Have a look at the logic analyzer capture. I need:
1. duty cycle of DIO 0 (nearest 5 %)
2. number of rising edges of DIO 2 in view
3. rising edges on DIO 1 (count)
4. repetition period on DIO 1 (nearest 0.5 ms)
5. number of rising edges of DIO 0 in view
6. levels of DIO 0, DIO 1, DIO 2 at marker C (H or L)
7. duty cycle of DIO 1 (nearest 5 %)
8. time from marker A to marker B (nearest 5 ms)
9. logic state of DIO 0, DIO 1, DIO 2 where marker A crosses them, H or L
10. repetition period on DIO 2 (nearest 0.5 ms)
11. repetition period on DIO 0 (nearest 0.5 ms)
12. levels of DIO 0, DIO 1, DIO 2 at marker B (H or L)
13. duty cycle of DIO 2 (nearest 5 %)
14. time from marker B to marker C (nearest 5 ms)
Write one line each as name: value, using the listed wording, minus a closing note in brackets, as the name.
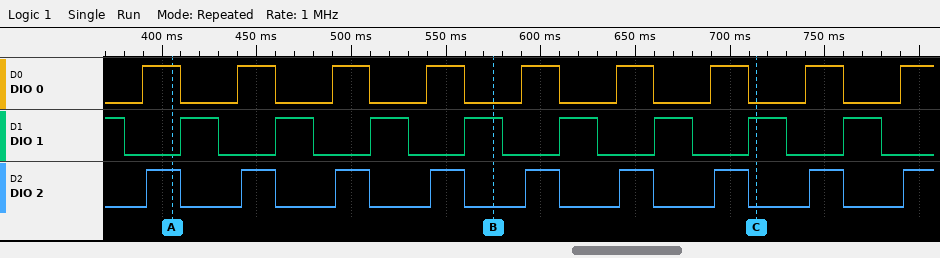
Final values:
duty cycle of DIO 0: 40 %
number of rising edges of DIO 2 in view: 9
rising edges on DIO 1: 8
repetition period on DIO 1: 50 ms
number of rising edges of DIO 0 in view: 9
levels of DIO 0, DIO 1, DIO 2 at marker C: DIO 0=L, DIO 1=H, DIO 2=L
duty cycle of DIO 1: 40 %
time from marker A to marker B: 170 ms
logic state of DIO 0, DIO 1, DIO 2 where marker A crosses them, H or L: DIO 0=H, DIO 1=L, DIO 2=H
repetition period on DIO 2: 50 ms
repetition period on DIO 0: 50 ms
levels of DIO 0, DIO 1, DIO 2 at marker B: DIO 0=L, DIO 1=H, DIO 2=L
duty cycle of DIO 2: 35 %
time from marker B to marker C: 140 ms
